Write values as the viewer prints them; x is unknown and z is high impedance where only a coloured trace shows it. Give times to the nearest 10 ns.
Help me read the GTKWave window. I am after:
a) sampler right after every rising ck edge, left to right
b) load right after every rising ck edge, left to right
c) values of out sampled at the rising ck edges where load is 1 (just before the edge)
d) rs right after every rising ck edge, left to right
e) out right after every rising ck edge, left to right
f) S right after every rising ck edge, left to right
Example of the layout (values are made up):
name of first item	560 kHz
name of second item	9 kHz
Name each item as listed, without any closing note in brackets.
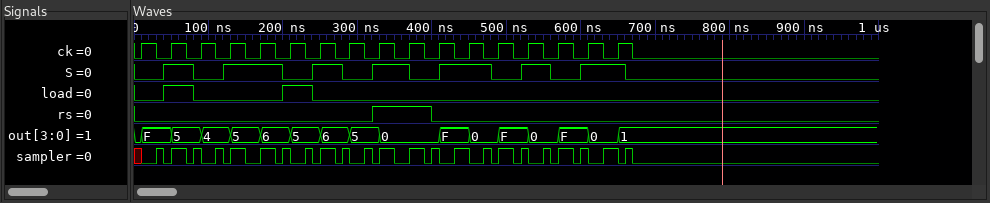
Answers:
sampler right after every rising ck edge, left to right	0 1 0 1 1 0 1 0 1 1 0 0 1 0 1 0 0
load right after every rising ck edge, left to right	0 1 0 0 0 1 0 0 0 0 0 0 0 0 0 0 0
values of out sampled at the rising ck edges where load is 1	F, 6
rs right after every rising ck edge, left to right	0 0 0 0 0 0 0 0 1 1 0 0 0 0 0 0 0
out right after every rising ck edge, left to right	F, 5, 4, 5, 6, 5, 6, 5, 0, 0, F, 0, F, 0, F, 0, 1
S right after every rising ck edge, left to right	0 1 0 1 1 0 1 0 1 0 1 1 0 1 0 1 1
